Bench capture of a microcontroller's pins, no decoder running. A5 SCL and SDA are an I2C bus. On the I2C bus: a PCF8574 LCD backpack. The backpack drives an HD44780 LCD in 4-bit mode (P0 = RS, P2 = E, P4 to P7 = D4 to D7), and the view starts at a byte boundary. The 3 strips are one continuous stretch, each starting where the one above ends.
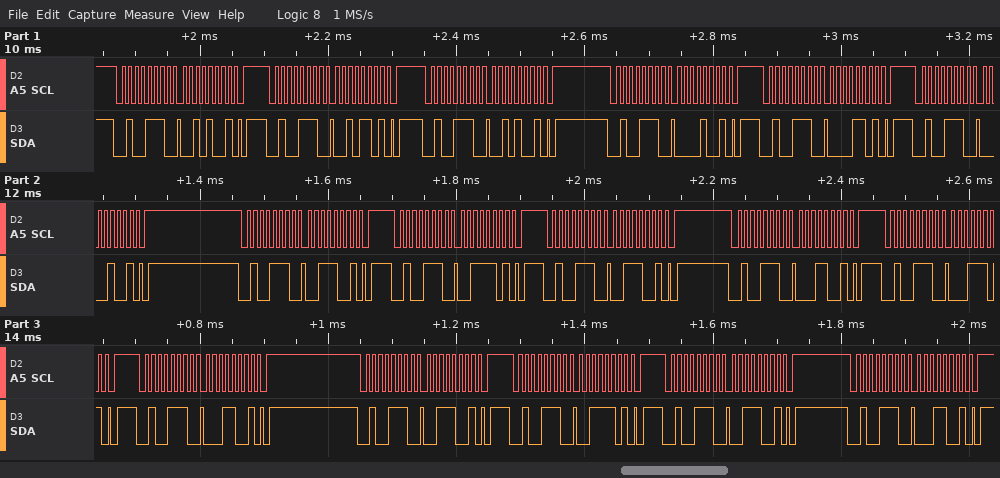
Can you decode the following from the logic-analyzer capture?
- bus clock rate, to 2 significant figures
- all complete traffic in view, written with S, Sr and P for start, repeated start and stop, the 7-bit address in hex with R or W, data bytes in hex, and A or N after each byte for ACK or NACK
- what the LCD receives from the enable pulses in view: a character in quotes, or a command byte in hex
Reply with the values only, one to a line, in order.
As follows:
100 kHz
S 27W A 29 A P S 27W A 2D A P S 27W A 29 A P S 27W A 09 A P S 27W A 0D A P S 27W A 09 A P S 27W A 39 A P S 27W A 3D A P S 27W A 39 A P S 27W A 19 A P S 27W A 1D A P S 27W A 19 A P S 27W A 39 A P S 27W A 3D A P S 27W A 39 A P S 27W A 19 A P
' ' '1'
